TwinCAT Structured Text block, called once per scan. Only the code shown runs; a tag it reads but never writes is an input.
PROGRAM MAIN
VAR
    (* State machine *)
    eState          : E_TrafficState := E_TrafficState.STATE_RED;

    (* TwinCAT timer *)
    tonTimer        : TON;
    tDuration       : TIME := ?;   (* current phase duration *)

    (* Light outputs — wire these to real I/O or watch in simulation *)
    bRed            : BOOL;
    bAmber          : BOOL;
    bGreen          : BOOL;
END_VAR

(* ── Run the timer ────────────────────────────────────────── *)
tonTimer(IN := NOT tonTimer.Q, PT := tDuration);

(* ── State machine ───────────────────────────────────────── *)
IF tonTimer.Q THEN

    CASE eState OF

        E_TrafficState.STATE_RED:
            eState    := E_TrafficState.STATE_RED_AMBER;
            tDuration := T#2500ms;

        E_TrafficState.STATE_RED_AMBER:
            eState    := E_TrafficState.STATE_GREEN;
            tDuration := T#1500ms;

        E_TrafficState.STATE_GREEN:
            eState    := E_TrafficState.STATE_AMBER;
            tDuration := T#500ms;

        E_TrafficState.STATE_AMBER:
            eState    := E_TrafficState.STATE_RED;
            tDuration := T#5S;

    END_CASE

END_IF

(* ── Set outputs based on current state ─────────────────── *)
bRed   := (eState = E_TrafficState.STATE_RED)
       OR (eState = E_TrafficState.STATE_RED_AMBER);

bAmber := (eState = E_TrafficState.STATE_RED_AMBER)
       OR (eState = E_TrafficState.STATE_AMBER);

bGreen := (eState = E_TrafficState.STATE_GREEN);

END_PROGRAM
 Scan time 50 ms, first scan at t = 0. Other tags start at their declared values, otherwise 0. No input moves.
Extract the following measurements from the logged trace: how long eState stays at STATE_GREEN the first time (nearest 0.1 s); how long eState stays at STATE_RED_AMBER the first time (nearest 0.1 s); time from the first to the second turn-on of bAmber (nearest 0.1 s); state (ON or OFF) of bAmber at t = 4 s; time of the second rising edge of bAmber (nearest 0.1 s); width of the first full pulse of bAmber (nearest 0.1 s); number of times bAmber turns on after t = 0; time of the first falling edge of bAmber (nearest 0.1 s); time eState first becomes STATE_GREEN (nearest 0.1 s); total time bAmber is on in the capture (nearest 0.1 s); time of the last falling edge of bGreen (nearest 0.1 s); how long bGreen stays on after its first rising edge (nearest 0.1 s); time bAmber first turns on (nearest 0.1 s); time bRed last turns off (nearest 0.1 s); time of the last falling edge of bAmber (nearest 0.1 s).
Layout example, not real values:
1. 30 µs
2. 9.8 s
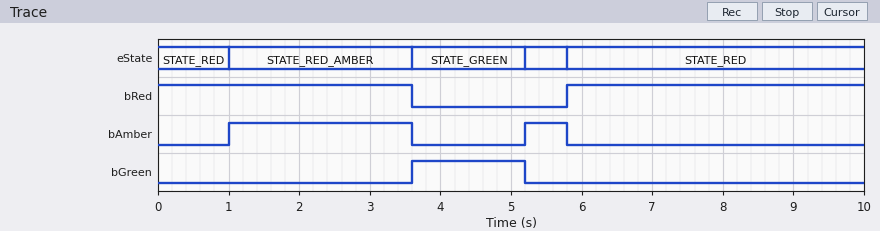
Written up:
1. 1.6 s
2. 2.6 s
3. 4.2 s
4. OFF
5. 5.2 s
6. 2.6 s
7. 2
8. 3.6 s
9. 3.6 s
10. 3.2 s
11. 5.2 s
12. 1.6 s
13. 1.0 s
14. 3.6 s
15. 5.8 s
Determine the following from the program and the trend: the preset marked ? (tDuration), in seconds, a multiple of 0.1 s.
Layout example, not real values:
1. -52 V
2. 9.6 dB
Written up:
1. 1.0 s
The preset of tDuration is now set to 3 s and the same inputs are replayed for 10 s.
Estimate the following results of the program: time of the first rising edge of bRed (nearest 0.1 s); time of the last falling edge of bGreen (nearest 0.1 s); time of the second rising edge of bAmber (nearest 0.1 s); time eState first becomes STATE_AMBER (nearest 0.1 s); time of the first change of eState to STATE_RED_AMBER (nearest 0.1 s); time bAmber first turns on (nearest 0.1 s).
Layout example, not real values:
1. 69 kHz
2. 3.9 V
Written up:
1. 7.8 s
2. 7.2 s
3. 7.2 s
4. 7.2 s
5. 3.0 s
6. 3.0 s
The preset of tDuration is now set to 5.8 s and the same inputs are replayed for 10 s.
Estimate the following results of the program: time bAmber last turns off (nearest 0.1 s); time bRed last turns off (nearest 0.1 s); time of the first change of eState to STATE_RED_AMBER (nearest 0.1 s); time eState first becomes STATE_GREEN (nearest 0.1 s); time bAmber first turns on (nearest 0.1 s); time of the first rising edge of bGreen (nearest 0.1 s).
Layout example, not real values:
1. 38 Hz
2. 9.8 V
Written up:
1. 8.4 s
2. 8.4 s
3. 5.8 s
4. 8.4 s
5. 5.8 s
6. 8.4 s
